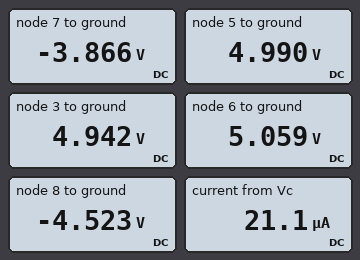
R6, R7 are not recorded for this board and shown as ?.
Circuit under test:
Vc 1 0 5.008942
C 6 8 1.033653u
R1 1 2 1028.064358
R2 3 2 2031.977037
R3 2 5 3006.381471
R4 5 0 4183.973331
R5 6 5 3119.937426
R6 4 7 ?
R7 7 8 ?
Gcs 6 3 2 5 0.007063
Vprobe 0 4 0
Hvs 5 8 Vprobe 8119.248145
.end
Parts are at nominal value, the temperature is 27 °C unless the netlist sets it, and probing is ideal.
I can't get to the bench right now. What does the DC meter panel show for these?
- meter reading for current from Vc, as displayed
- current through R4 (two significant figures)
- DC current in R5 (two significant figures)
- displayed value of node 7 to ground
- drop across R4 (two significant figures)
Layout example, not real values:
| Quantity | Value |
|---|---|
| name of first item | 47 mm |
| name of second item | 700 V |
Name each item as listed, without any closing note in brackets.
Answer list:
| Quantity | Value |
|---|---|
| meter reading for current from Vc, as displayed | 21.1 µA |
| current through R4 | 1.2 mA |
| DC current in R5 | 22 µA |
| displayed value of node 7 to ground | -3.866 V |
| drop across R4 | 5.0 V |
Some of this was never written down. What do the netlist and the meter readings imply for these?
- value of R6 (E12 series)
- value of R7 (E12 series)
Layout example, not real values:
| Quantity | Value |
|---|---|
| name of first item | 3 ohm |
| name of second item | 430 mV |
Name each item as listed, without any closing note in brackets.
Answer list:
| Quantity | Value |
|---|---|
| value of R6 | 3.3 kΩ |
| value of R7 | 560 Ω |
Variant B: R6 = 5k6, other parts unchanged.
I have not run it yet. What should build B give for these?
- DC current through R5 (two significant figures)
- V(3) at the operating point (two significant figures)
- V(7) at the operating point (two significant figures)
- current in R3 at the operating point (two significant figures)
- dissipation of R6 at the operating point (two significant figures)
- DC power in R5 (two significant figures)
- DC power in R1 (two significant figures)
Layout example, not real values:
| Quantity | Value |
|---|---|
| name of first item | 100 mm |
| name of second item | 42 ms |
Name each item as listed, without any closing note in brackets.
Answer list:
| Quantity | Value |
|---|---|
| DC current through R5 | 1.9 mA |
| V(3) at the operating point | 11 V |
| V(7) at the operating point | -19 V |
| current in R3 at the operating point | 88 µA |
| dissipation of R6 at the operating point | 63 mW |
| DC power in R5 | 11 mW |
| DC power in R1 | 3.3 mW |
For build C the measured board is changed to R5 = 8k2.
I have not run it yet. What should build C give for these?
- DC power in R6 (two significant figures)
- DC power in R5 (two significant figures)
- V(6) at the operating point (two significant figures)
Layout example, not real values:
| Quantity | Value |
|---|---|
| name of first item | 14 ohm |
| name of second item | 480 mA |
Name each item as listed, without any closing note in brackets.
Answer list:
| Quantity | Value |
|---|---|
| DC power in R6 | 4.5 mW |
| DC power in R5 | 4.0 µW |
| V(6) at the operating point | 5.2 V |
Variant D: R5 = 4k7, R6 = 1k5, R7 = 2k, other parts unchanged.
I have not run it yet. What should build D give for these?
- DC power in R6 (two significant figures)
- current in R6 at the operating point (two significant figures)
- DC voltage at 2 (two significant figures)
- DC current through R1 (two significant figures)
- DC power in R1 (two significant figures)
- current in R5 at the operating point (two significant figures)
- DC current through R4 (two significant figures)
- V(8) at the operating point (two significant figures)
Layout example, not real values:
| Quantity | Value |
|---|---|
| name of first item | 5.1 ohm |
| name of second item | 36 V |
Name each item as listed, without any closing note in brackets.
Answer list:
| Quantity | Value |
|---|---|
| DC power in R6 | 1.7 mW |
| current in R6 at the operating point | 1.1 mA |
| DC voltage at 2 | 4.9 V |
| DC current through R1 | 110 µA |
| DC power in R1 | 13 µW |
| current in R5 at the operating point | 120 µA |
| DC current through R4 | 1.2 mA |
| V(8) at the operating point | -3.7 V |
